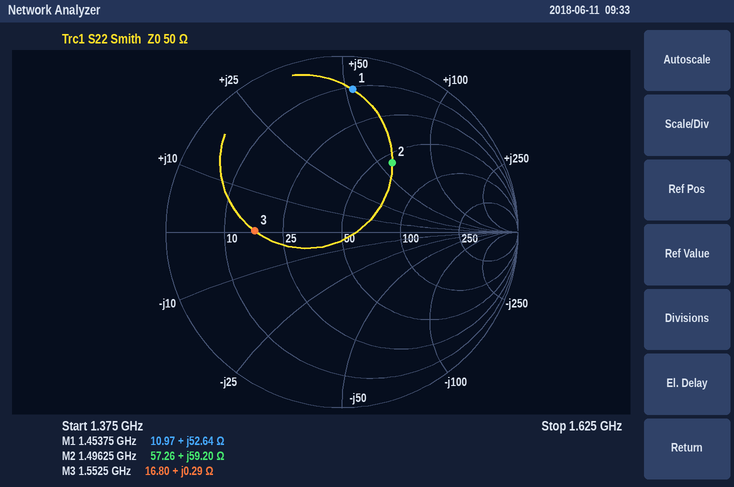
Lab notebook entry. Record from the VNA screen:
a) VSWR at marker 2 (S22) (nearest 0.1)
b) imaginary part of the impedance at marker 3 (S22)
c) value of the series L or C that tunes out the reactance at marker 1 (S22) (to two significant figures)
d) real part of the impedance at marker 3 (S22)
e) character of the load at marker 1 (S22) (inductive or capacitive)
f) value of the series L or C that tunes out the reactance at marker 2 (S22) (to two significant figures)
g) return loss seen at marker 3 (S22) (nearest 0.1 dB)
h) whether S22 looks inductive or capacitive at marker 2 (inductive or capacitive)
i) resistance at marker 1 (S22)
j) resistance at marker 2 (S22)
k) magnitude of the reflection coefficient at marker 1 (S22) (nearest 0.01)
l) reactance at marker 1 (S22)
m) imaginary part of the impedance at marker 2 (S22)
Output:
2.9
+0.29 Ω
2.1 pF
16.80 Ω
inductive
1.8 pF
6.1 dB
inductive
10.97 Ω
57.26 Ω
0.81
+52.64 Ω
+59.20 Ω
